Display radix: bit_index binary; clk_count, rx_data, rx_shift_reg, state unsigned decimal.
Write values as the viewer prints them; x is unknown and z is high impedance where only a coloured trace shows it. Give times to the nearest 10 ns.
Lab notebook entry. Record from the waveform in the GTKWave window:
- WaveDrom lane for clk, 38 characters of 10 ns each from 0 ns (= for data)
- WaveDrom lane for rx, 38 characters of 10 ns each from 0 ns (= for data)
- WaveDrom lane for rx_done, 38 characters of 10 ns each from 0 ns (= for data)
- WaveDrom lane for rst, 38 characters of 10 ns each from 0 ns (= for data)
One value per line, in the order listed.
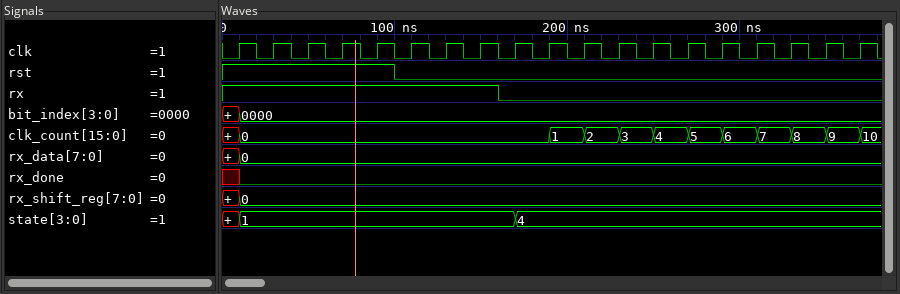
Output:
{name: 'clk', wave: '01010101010101010101010101010101010101'}
{name: 'rx', wave: '1...............0.....................'}
{name: 'rx_done', wave: 'x0....................................'}
{name: 'rst', wave: '1.........0...........................'}
